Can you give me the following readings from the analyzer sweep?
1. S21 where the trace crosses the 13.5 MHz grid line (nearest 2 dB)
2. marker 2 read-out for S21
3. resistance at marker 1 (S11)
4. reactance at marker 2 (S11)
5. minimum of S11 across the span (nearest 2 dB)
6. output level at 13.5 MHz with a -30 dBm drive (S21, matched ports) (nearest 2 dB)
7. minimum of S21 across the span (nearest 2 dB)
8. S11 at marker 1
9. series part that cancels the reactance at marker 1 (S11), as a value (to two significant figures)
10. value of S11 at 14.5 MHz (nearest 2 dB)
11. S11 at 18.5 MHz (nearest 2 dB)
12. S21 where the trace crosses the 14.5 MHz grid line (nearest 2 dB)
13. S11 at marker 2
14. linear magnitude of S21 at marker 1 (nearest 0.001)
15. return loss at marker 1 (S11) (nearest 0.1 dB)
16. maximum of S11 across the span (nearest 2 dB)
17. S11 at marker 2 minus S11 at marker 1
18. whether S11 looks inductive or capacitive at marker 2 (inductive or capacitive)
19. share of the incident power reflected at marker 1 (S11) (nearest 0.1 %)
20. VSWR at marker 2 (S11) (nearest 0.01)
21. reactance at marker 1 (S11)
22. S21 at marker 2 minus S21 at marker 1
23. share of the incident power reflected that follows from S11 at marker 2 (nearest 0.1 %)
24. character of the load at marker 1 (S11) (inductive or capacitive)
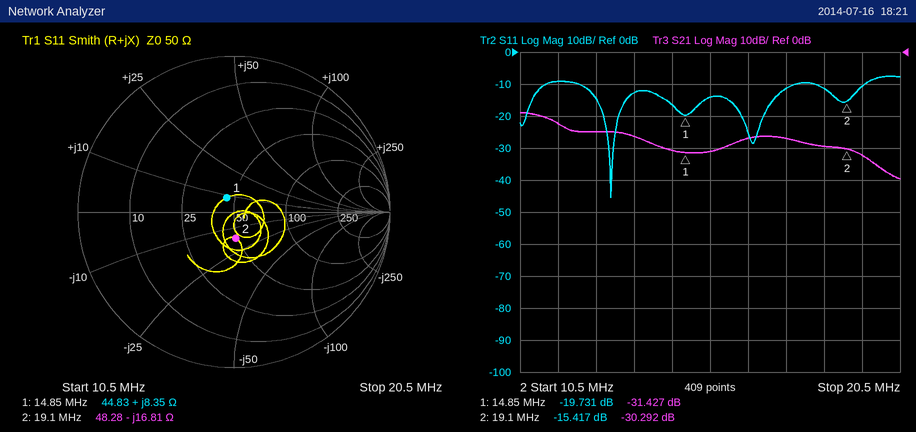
-26 dB
-30.292 dB
44.83 Ω
-16.81 Ω
-46 dB
-56 dBm
-40 dB
-19.731 dB
1.3 nF
-16 dB
-12 dB
-30 dB
-15.417 dB
0.027
19.7 dB
-8 dB
4.314 dB
capacitive
1.1 %
1.41
+8.35 Ω
1.135 dB
2.9 %
inductive
